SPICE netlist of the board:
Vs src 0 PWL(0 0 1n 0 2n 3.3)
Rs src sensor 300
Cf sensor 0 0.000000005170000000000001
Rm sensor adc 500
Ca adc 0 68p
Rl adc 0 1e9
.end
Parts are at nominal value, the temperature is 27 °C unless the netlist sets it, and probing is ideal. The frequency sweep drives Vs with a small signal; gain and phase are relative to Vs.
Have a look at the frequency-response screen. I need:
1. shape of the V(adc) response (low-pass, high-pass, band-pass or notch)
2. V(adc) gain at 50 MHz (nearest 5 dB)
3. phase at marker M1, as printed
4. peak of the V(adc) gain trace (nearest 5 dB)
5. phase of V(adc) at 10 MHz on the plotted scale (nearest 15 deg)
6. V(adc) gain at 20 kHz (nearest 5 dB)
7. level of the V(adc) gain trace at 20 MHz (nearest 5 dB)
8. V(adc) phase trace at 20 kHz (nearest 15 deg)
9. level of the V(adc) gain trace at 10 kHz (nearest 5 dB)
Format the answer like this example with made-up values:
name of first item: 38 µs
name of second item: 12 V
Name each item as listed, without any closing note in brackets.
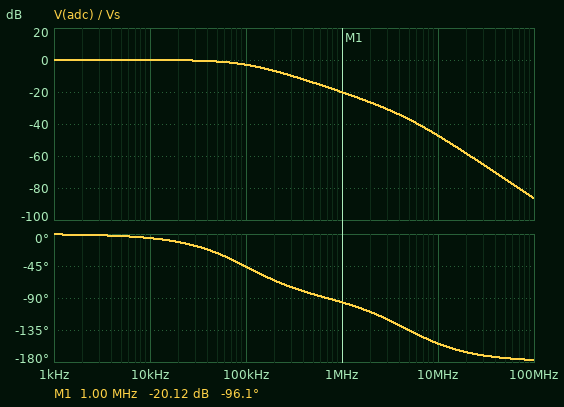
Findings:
shape of the V(adc) response: low-pass
V(adc) gain at 50 MHz: -75 dB
phase at marker M1, as printed: -96.1 deg
peak of the V(adc) gain trace: 0 dB
phase of V(adc) at 10 MHz on the plotted scale: -150 deg
V(adc) gain at 20 kHz: 0 dB
level of the V(adc) gain trace at 20 MHz: -60 dB
V(adc) phase trace at 20 kHz: -15 deg
level of the V(adc) gain trace at 10 kHz: 0 dB
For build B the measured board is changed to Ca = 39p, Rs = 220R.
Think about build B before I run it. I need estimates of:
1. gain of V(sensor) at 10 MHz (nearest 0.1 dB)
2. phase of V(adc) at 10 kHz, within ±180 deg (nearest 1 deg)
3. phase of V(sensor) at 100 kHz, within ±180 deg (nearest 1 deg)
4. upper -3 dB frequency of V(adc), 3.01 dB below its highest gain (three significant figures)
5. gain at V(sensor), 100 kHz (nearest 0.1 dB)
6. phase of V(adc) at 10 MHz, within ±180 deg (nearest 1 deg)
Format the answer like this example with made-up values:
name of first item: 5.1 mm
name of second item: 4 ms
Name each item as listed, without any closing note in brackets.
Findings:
gain of V(sensor) at 10 MHz: -37.1 dB
phase of V(adc) at 10 kHz, within ±180 deg: -4 deg
phase of V(sensor) at 100 kHz, within ±180 deg: -36 deg
upper -3 dB frequency of V(adc), 3.01 dB below its highest gain: 139 kHz
gain at V(sensor), 100 kHz: -1.8 dB
phase of V(adc) at 10 MHz, within ±180 deg: -140 deg
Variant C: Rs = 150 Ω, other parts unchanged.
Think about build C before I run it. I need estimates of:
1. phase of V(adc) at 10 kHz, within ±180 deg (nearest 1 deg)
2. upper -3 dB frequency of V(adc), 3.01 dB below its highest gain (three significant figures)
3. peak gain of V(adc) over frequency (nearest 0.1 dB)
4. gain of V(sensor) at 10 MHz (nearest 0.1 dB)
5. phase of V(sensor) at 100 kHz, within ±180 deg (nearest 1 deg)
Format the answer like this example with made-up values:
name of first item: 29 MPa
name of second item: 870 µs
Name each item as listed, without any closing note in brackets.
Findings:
phase of V(adc) at 10 kHz, within ±180 deg: -3 deg
upper -3 dB frequency of V(adc), 3.01 dB below its highest gain: 202 kHz
peak gain of V(adc) over frequency: 0 dB
gain of V(sensor) at 10 MHz: -33.8 dB
phase of V(sensor) at 100 kHz, within ±180 deg: -26 deg
